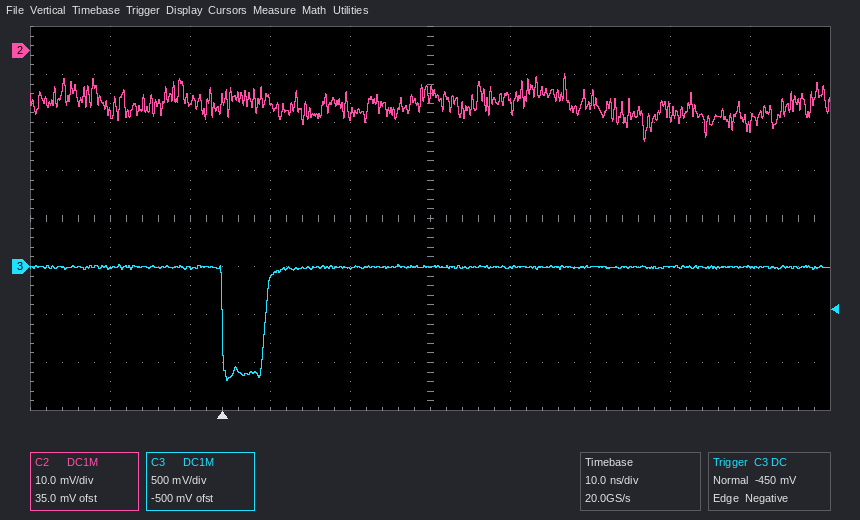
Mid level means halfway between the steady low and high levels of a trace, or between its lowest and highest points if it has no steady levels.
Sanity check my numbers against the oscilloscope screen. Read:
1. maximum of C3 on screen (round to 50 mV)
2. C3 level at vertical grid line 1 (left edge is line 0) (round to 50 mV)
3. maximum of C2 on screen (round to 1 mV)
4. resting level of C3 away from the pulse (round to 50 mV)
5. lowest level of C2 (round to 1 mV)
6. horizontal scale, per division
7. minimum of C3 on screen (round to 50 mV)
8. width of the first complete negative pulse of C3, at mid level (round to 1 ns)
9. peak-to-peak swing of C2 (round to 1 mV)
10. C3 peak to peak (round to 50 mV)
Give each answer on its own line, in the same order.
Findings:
0 mV
0 mV
-5 mV
0 mV
-19 mV
10 ns
-1.20 V
5 ns
14 mV
1.20 V
